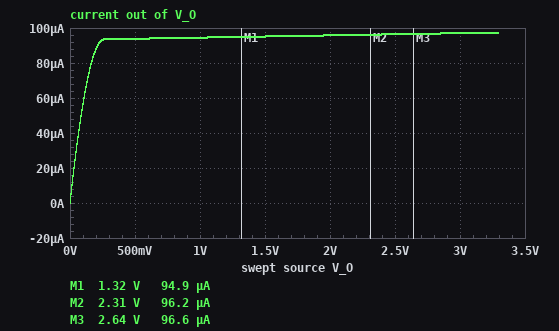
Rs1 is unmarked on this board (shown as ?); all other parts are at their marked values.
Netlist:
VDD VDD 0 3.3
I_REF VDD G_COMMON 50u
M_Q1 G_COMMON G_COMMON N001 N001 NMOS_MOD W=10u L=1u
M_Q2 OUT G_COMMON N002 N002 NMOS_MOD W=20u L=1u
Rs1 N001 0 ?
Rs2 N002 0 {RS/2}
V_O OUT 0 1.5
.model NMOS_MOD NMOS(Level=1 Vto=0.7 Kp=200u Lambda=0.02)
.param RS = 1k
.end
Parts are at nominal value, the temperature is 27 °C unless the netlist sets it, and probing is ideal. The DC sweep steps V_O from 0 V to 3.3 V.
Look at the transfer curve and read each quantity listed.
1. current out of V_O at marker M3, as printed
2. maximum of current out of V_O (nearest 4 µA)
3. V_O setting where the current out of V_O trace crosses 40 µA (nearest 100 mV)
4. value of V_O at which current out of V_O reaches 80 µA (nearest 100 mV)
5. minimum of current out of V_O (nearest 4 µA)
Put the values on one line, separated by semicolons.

96.6 µA; 96 µA; 100 mV; 200 mV; 0 A
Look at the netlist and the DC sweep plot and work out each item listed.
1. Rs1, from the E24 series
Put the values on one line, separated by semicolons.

820 Ω
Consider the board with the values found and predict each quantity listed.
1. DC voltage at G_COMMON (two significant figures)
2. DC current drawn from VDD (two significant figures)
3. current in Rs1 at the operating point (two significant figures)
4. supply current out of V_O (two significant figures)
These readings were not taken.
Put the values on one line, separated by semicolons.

960 mV; 50 µA; 50 µA; 95 µA
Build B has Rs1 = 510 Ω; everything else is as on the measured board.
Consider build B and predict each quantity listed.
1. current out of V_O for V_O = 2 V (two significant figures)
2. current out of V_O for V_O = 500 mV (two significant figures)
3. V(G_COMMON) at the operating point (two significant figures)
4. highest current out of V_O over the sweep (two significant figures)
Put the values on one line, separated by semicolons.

86 µA; 85 µA; 950 mV; 88 µA
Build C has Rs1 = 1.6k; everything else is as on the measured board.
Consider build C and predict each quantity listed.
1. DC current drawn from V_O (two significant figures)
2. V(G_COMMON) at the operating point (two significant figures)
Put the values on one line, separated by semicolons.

120 µA; 1.0 V
